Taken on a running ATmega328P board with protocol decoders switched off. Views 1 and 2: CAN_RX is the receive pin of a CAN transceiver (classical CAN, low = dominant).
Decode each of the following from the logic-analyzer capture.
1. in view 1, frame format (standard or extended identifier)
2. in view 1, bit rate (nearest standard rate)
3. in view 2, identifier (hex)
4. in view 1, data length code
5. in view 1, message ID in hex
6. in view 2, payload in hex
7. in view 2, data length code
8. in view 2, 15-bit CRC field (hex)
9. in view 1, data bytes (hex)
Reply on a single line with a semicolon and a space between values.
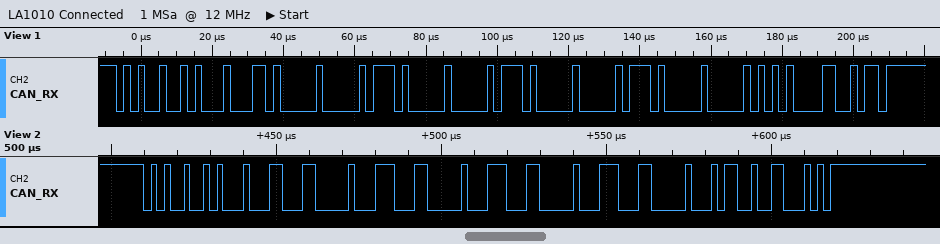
standard; 500 kbit/s; 0x525; 8; 0x525; C6 01 C6 01 C6 01 C6 01; 8; 0x3262; D0 01 D0 01 D0 01 D0 01
